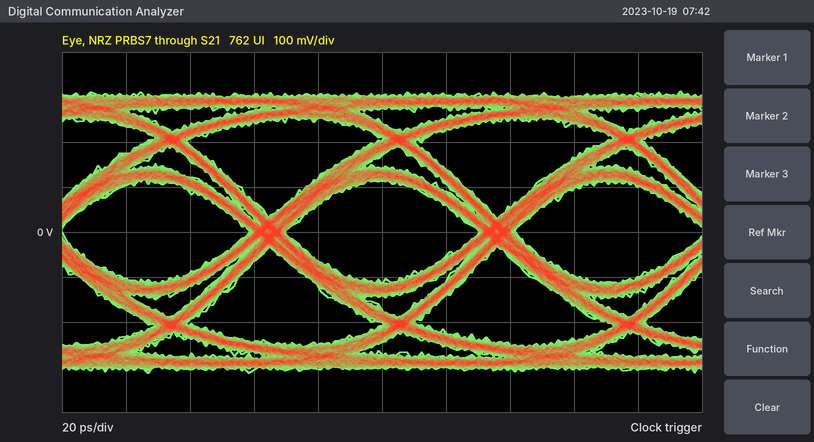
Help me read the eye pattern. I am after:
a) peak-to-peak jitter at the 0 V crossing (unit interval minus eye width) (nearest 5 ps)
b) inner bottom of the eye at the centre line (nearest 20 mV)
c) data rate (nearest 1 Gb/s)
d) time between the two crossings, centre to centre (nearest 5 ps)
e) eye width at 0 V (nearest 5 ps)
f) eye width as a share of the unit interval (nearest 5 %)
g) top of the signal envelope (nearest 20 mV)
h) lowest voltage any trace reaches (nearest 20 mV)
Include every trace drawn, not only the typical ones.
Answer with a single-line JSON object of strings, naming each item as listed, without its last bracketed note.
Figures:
{"peak-to-peak jitter at the 0 V crossing (unit interval minus eye width)": "10 ps", "inner bottom of the eye at the centre line": "-120 mV", "data rate": "14 Gb/s", "time between the two crossings, centre to centre": "70 ps", "eye width at 0 V": "60 ps", "eye width as a share of the unit interval": "85 %", "top of the signal envelope": "320 mV", "lowest voltage any trace reaches": "-320 mV"}
